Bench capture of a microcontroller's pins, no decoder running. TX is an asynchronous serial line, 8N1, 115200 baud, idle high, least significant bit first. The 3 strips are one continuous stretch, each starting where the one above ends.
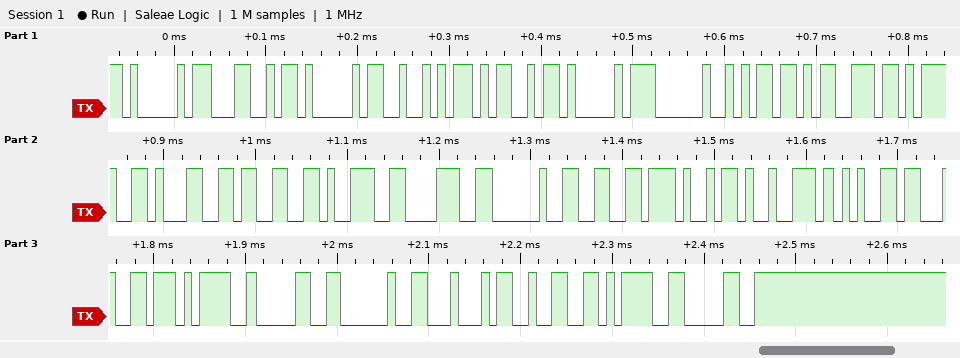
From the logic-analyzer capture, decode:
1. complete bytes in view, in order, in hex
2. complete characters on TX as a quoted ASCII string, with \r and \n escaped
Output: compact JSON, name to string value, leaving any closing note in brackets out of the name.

{"complete bytes in view, in order, in hex": "41 4C 41 52 4D 41 20 6D 73 3D 31 33 39 38 20 66 69 72 65 64 3D 30 20 44 32 3D 30", "complete characters on TX as a quoted ASCII string, with \\r and \\n escaped": "\"ALARMA ms=1398 fired=0 D2=0\""}
